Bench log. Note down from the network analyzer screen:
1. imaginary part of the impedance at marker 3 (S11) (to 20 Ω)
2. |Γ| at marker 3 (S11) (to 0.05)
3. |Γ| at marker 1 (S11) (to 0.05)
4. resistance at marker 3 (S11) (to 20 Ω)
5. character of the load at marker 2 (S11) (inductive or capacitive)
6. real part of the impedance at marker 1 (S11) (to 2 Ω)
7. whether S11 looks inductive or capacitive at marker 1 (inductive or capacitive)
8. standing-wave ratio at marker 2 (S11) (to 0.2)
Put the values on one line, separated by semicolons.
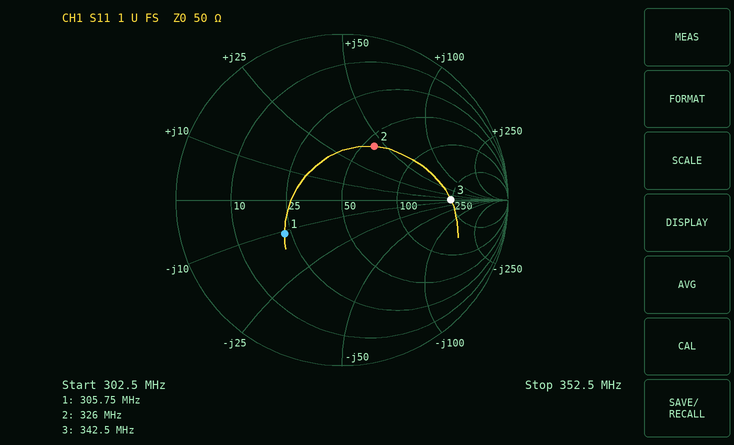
0 Ω; 0.65; 0.40; 240 Ω; inductive; 22 Ω; capacitive; 2.2
